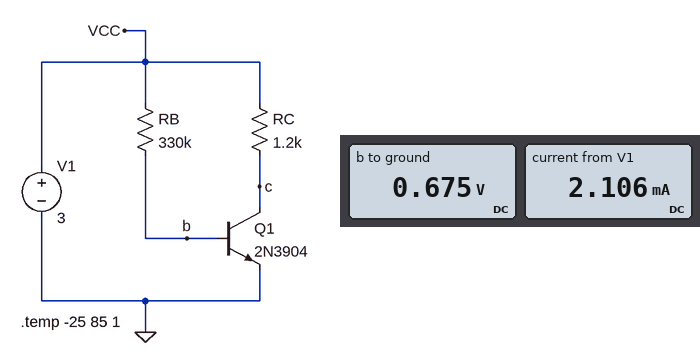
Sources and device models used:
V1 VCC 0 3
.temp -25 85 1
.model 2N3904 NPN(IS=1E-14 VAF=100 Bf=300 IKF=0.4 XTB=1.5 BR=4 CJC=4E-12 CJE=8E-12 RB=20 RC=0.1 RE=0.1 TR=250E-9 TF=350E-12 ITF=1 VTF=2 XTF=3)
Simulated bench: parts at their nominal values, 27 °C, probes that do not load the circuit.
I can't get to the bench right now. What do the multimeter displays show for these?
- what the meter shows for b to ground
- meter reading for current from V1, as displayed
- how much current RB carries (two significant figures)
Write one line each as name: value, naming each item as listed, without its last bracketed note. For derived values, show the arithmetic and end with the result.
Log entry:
what the meter shows for b to ground: 0.675 V
meter reading for current from V1, as displayed: 2.106 mA
how much current RB carries: (3 V - 675 mV) / 330 kΩ = 7.0 µA
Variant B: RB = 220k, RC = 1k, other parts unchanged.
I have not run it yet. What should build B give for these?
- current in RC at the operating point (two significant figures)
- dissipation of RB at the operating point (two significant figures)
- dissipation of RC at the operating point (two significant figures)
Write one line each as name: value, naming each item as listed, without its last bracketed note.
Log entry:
current in RC at the operating point: 2.8 mA
dissipation of RB at the operating point: 24 µW
dissipation of RC at the operating point: 8.0 mW
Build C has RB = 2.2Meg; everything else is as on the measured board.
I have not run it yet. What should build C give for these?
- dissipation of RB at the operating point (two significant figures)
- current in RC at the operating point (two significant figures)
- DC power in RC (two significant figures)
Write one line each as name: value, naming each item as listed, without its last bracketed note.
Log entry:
dissipation of RB at the operating point: 2.6 µW
current in RC at the operating point: 330 µA
DC power in RC: 130 µW
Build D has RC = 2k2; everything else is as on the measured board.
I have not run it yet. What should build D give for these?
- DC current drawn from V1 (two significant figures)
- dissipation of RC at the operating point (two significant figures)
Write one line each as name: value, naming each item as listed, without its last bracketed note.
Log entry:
DC current drawn from V1: 1.3 mA
dissipation of RC at the operating point: 3.8 mW
